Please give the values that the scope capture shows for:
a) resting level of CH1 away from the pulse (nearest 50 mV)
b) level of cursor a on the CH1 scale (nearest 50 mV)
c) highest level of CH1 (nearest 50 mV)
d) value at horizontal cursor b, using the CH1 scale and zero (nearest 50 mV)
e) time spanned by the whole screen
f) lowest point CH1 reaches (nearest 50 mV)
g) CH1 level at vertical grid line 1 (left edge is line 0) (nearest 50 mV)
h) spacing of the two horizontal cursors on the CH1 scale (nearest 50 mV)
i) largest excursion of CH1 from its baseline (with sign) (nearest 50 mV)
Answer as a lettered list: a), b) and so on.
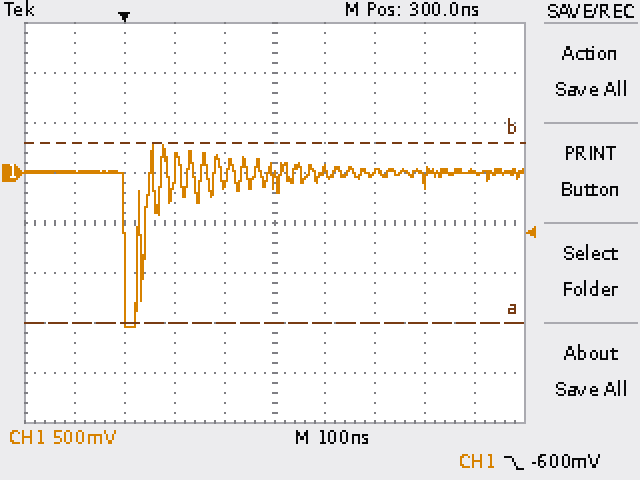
a) 0 mV
b) -1.50 V
c) 300 mV
d) 300 mV
e) 1 µs
f) -1.55 V
g) 0 mV
h) 1.80 V
i) -1.55 V
